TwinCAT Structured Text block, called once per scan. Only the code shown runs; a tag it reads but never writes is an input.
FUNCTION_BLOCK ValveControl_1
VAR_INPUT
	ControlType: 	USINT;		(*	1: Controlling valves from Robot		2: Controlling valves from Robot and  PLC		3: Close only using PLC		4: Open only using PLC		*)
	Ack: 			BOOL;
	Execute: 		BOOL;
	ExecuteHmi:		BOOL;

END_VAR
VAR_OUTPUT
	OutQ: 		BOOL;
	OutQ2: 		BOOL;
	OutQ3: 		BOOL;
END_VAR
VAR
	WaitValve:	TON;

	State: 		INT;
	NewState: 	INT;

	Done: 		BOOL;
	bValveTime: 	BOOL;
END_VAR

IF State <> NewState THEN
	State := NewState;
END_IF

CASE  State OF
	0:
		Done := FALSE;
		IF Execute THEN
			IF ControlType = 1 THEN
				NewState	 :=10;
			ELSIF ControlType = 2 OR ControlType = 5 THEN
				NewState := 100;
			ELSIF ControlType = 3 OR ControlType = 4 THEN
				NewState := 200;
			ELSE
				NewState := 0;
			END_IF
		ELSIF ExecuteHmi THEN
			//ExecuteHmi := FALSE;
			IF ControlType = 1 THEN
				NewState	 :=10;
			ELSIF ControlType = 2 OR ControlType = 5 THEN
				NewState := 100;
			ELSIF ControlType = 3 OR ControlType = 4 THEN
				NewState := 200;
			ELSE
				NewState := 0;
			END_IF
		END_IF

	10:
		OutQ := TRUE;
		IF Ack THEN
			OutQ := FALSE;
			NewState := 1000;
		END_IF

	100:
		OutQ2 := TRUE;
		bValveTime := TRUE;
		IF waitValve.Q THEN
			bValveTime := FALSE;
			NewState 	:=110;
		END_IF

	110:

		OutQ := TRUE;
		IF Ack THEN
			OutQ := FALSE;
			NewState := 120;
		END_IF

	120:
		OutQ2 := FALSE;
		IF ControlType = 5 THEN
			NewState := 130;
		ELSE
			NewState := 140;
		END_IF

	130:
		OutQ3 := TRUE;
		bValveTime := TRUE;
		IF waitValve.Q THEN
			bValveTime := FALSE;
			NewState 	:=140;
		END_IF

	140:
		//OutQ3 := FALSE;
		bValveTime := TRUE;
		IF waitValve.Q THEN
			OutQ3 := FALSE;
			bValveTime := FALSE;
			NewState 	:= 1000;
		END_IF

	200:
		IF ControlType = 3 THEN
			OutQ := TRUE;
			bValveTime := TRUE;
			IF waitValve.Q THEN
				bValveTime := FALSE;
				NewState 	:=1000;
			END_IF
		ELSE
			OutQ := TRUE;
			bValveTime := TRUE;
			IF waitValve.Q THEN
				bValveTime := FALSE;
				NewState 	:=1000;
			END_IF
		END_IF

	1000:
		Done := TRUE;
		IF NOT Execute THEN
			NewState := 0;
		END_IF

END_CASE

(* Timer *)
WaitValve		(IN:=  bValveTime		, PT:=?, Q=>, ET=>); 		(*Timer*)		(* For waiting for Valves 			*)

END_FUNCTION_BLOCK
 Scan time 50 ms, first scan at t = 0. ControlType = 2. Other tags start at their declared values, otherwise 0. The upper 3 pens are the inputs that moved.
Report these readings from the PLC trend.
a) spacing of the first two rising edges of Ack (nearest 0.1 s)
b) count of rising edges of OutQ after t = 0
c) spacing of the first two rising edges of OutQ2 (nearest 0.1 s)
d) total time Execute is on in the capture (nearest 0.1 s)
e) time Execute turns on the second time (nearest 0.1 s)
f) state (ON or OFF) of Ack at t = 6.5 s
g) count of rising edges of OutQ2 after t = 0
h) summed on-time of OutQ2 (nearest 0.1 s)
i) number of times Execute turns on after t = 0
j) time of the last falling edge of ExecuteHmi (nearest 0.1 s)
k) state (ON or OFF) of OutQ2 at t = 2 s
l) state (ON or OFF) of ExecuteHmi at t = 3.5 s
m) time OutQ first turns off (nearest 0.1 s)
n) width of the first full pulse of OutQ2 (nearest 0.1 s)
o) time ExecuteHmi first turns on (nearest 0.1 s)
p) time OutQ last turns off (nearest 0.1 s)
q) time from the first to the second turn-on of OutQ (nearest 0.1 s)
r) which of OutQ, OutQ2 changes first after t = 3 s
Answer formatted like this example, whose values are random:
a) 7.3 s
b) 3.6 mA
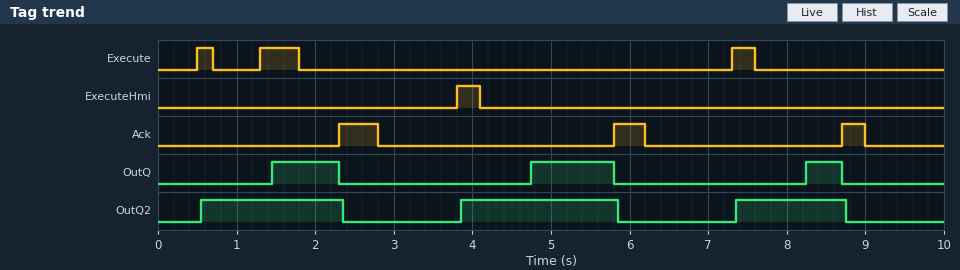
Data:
a) 3.5 s
b) 3
c) 3.3 s
d) 1.0 s
e) 1.3 s
f) OFF
g) 3
h) 5.2 s
i) 3
j) 4.1 s
k) ON
l) OFF
m) 2.3 s
n) 1.8 s
o) 3.8 s
p) 8.7 s
q) 3.3 s
r) OutQ2
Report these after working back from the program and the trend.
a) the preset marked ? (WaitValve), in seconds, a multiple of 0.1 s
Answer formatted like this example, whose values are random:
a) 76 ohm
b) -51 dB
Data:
a) 0.8 s
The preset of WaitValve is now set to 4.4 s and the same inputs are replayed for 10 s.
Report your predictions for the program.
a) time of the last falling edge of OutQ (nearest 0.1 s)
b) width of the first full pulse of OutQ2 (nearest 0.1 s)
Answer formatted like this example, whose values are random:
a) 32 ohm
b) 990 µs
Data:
a) 5.8 s
b) 5.3 s
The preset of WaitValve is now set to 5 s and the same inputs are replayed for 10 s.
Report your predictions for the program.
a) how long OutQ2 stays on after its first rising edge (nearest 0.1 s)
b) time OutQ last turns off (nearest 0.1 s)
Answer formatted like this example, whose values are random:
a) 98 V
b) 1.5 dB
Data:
a) 5.3 s
b) 5.8 s
